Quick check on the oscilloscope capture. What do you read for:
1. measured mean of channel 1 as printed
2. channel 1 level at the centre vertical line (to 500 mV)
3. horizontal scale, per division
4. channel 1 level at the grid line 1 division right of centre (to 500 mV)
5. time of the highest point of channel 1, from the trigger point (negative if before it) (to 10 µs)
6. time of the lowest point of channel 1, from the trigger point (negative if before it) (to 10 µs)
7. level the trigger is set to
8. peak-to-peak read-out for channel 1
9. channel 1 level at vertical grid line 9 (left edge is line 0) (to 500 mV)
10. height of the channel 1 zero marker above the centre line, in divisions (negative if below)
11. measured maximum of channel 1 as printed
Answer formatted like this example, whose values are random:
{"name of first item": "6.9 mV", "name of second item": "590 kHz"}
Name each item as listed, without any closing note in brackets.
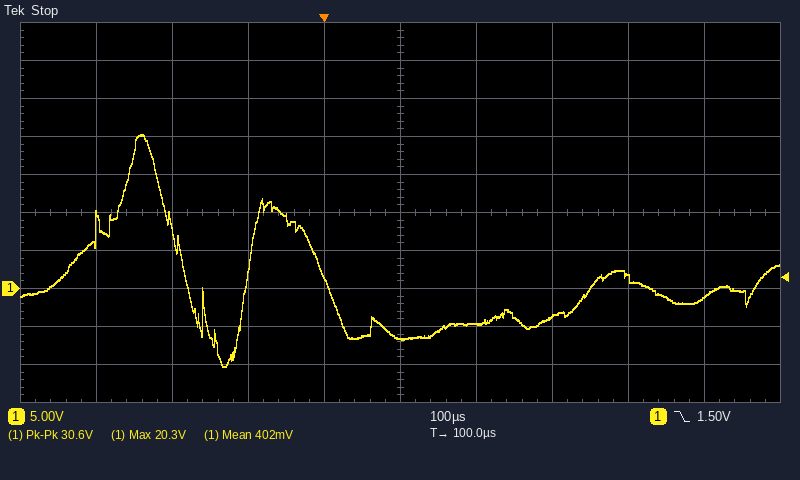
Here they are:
{"measured mean of channel 1 as printed": "402 mV", "channel 1 level at the centre vertical line": "-6.5 V", "horizontal scale, per division": "100 µs", "channel 1 level at the grid line 1 division right of centre": "-4.5 V", "time of the highest point of channel 1, from the trigger point (negative if before it)": "-240 µs", "time of the lowest point of channel 1, from the trigger point (negative if before it)": "-130 µs", "level the trigger is set to": "1.50 V", "peak-to-peak read-out for channel 1": "30.6 V", "channel 1 level at vertical grid line 9 (left edge is line 0)": "-1.0 V", "height of the channel 1 zero marker above the centre line, in divisions": "-2.0 div", "measured maximum of channel 1 as printed": "20.3 V"}
